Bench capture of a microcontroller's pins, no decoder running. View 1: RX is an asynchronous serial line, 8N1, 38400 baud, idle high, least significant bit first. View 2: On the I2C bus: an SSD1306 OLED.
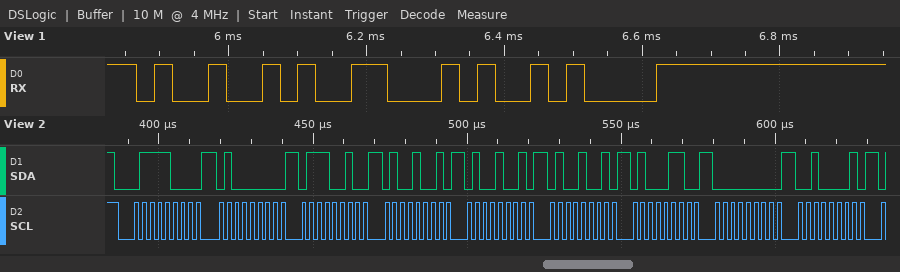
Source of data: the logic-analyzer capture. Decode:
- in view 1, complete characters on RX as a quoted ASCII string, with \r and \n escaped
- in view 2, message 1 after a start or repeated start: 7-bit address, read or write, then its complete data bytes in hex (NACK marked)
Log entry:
"IF\n"
0x3C write: 40 72 49 49 49 46 00 21
